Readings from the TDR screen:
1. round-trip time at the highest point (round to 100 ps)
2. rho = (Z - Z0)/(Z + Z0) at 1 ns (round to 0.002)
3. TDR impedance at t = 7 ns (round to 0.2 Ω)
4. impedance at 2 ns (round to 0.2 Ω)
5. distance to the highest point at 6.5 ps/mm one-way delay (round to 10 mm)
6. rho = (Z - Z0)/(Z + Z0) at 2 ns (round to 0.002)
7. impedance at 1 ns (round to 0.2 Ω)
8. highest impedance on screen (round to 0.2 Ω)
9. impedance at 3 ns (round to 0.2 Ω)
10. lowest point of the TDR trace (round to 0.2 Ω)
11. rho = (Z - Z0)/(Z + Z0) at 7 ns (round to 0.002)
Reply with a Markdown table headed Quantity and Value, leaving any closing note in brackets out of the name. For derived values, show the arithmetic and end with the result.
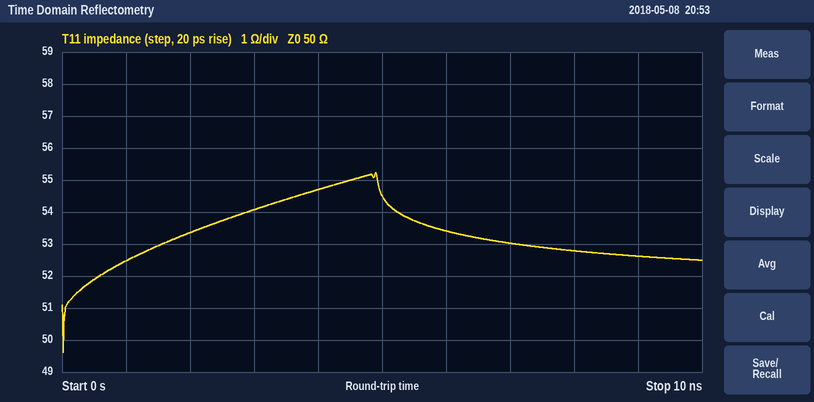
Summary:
| Quantity | Value |
|---|---|
| round-trip time at the highest point | 4.9 ns |
| rho = (Z - Z0)/(Z + Z0) at 1 ns | (52.4 − 50)/(52.4 + 50) ≈ +0.0234, so +0.024 to the nearest 0.002 |
| TDR impedance at t = 7 ns | 53.0 Ω |
| impedance at 2 ns | 53.4 Ω |
| distance to the highest point at 6.5 ps/mm one-way delay | 4.9 ns / 2 / 6.5 ps/mm ≈ 377 mm, so 380 mm to the nearest 10 mm |
| rho = (Z - Z0)/(Z + Z0) at 2 ns | (53.4 − 50)/(53.4 + 50) ≈ +0.0329, so +0.032 to the nearest 0.002 |
| impedance at 1 ns | 52.4 Ω |
| highest impedance on screen | 55.2 Ω |
| impedance at 3 ns | 54.0 Ω |
| lowest point of the TDR trace | 49.6 Ω |
| rho = (Z - Z0)/(Z + Z0) at 7 ns | (53 − 50)/(53 + 50) ≈ +0.0291, so +0.030 to the nearest 0.002 |
